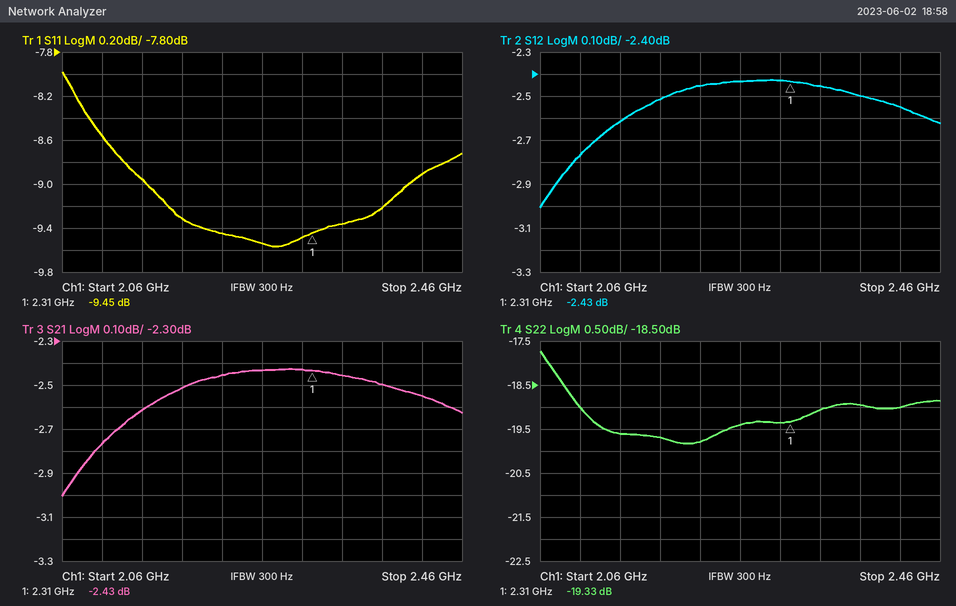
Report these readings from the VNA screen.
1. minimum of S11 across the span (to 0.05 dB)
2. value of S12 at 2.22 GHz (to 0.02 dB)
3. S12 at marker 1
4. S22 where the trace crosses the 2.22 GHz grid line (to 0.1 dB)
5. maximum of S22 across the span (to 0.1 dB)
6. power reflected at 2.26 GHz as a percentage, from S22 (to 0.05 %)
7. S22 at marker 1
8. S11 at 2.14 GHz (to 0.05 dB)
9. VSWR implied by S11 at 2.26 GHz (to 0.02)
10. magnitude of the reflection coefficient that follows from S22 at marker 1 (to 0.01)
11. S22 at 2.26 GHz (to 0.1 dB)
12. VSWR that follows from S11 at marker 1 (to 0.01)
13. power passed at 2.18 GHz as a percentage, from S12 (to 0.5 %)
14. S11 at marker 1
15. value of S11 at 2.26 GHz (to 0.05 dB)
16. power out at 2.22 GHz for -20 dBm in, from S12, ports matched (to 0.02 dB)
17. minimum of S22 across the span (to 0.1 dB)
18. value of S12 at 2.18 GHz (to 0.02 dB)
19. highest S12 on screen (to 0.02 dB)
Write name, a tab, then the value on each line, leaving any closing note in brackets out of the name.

minimum of S11 across the span	-9.55 dB
value of S12 at 2.22 GHz	-2.46 dB
S12 at marker 1	-2.43 dB
S22 where the trace crosses the 2.22 GHz grid line	-19.8 dB
maximum of S22 across the span	-17.7 dB
power reflected at 2.26 GHz as a percentage, from S22	1.15 %
S22 at marker 1	-19.33 dB
S11 at 2.14 GHz	-8.95 dB
VSWR implied by S11 at 2.26 GHz	2.00
magnitude of the reflection coefficient that follows from S22 at marker 1	0.11
S22 at 2.26 GHz	-19.4 dB
VSWR that follows from S11 at marker 1	2.02
power passed at 2.18 GHz as a percentage, from S12	56.0 %
S11 at marker 1	-9.45 dB
value of S11 at 2.26 GHz	-9.55 dB
power out at 2.22 GHz for -20 dBm in, from S12, ports matched	-22.46 dBm
minimum of S22 across the span	-19.8 dB
value of S12 at 2.18 GHz	-2.52 dB
highest S12 on screen	-2.42 dB
